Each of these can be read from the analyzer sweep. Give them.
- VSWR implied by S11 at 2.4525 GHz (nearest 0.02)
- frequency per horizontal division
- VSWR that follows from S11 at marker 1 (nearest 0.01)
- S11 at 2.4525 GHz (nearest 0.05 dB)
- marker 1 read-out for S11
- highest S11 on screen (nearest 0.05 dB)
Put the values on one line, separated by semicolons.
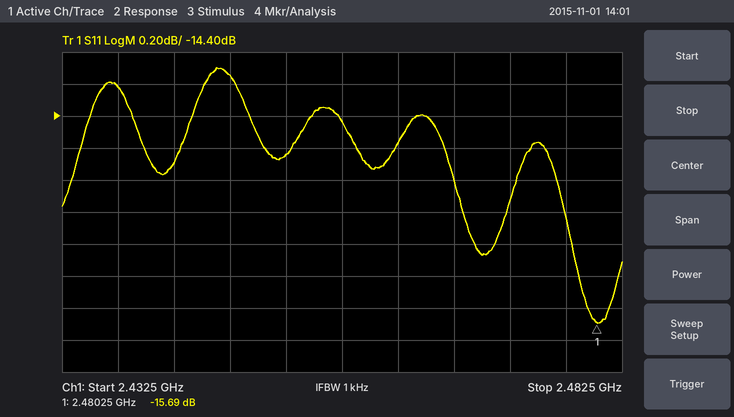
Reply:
1.46; 5 MHz; 1.39; -14.65 dB; -15.69 dB; -14.10 dB
